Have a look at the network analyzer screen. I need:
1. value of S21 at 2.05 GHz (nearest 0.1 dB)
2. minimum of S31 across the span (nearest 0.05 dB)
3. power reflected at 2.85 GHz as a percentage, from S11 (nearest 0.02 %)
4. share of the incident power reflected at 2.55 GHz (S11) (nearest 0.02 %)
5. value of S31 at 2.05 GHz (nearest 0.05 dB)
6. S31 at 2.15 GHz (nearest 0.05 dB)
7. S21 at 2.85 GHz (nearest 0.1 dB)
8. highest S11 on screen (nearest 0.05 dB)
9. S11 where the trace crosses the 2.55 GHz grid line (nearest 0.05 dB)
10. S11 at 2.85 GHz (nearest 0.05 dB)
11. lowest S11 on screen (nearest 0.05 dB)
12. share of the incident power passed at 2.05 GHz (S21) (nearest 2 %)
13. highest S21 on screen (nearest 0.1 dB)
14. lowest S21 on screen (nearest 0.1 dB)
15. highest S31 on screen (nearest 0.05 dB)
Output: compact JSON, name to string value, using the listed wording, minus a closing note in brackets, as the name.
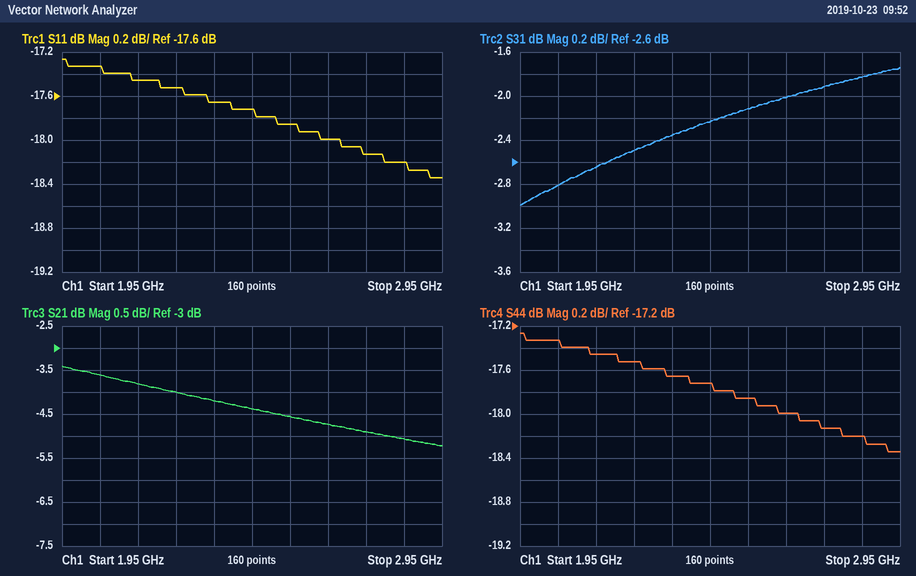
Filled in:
{"value of S21 at 2.05 GHz": "-3.6 dB", "minimum of S31 across the span": "-3.00 dB", "power reflected at 2.85 GHz as a percentage, from S11": "1.52 %", "share of the incident power reflected at 2.55 GHz (S11)": "1.64 %", "value of S31 at 2.05 GHz": "-2.80 dB", "S31 at 2.15 GHz": "-2.65 dB", "S21 at 2.85 GHz": "-5.1 dB", "highest S11 on screen": "-17.25 dB", "S11 where the trace crosses the 2.55 GHz grid line": "-17.85 dB", "S11 at 2.85 GHz": "-18.20 dB", "lowest S11 on screen": "-18.35 dB", "share of the incident power passed at 2.05 GHz (S21)": "44 %", "highest S21 on screen": "-3.4 dB", "lowest S21 on screen": "-5.2 dB", "highest S31 on screen": "-1.75 dB"}
